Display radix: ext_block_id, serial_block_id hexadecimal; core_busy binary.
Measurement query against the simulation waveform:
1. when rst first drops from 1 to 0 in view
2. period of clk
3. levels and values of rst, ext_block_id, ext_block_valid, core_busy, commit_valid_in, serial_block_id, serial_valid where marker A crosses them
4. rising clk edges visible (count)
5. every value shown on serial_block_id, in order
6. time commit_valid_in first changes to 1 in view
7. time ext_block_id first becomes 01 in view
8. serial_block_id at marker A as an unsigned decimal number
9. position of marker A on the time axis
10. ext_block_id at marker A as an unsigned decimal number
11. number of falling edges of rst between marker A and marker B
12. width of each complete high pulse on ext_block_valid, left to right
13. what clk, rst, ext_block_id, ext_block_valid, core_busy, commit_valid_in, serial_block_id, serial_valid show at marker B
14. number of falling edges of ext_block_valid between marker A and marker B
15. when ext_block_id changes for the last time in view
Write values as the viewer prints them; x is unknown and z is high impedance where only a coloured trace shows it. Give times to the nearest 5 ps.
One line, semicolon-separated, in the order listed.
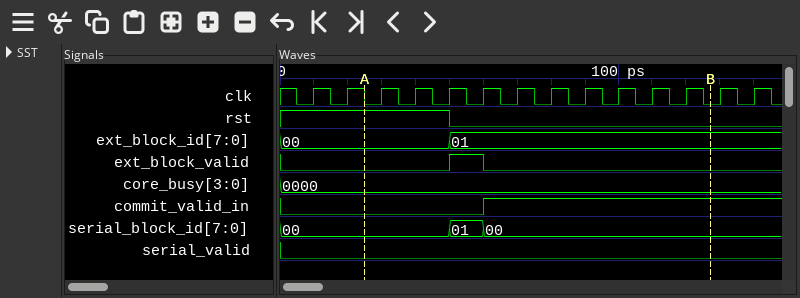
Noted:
50 ps; 10 ps; rst=1, ext_block_id=00, ext_block_valid=0, core_busy=0000, commit_valid_in=0, serial_block_id=00, serial_valid=0; 14; 00, 01, 00; 60 ps; 50 ps; 0; 25 ps; 0; 1; 10 ps; clk=0, rst=0, ext_block_id=01, ext_block_valid=0, core_busy=0000, commit_valid_in=1, serial_block_id=00, serial_valid=0; 1; 50 ps
